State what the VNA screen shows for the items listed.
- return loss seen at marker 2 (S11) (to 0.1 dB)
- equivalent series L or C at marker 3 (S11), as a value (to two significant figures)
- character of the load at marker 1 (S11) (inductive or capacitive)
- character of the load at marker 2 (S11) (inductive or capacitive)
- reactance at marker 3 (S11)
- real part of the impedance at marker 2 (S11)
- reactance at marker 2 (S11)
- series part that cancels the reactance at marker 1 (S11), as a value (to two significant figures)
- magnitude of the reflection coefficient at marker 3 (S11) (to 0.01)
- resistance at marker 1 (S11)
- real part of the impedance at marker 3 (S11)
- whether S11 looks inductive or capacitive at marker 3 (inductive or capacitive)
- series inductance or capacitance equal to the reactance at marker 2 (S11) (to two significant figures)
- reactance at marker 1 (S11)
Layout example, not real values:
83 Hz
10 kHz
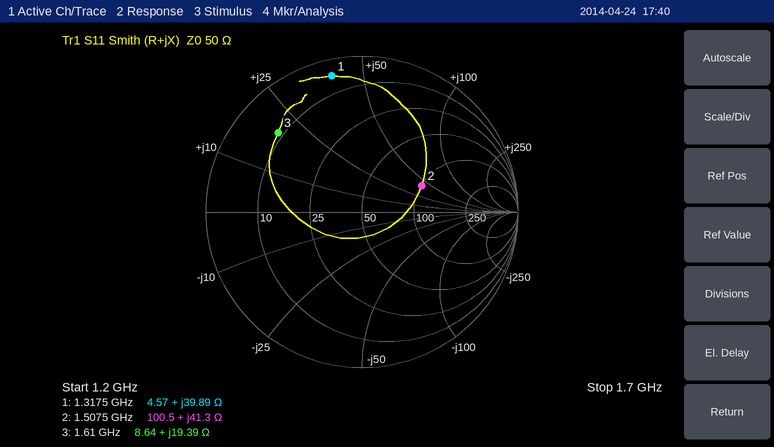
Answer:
7.6 dB
1.9 nH
inductive
inductive
+19.39 Ω
100.5 Ω
+41.3 Ω
3.0 pF
0.74
4.57 Ω
8.64 Ω
inductive
4.4 nH
+39.89 Ω
